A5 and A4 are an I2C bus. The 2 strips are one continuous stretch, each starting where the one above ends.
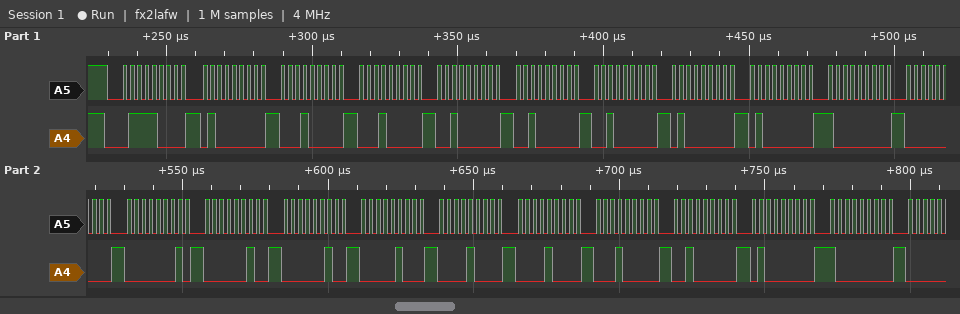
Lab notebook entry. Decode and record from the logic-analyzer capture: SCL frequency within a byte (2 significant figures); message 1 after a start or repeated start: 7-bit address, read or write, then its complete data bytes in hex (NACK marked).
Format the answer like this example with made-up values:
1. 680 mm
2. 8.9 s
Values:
1. 400 kHz
2. 0x3C write: 40 10 10 20 20 20 40 40 80 00 01 02 02 04 08 08 10 20 40 80
